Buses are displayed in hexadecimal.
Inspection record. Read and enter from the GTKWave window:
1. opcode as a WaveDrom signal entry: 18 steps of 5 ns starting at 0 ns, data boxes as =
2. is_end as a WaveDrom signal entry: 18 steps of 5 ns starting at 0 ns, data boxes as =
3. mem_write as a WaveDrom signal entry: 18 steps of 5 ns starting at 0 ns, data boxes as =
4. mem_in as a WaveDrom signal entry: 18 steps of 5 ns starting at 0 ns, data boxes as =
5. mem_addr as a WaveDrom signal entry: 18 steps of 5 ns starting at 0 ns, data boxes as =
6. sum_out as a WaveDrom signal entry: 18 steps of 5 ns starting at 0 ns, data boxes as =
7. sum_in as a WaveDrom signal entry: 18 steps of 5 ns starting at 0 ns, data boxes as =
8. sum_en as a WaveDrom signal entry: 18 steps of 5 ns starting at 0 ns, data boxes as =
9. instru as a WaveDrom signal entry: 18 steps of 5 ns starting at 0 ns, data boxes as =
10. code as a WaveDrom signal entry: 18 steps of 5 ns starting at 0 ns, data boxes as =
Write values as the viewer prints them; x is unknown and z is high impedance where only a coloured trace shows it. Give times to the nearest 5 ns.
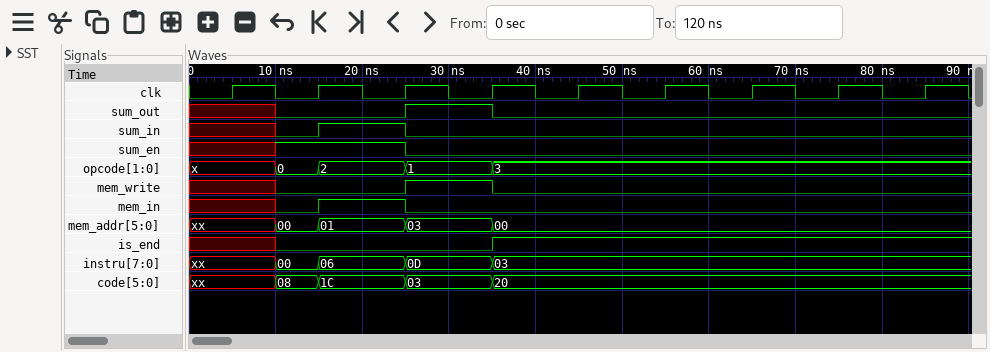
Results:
{name: 'opcode', wave: 'x.==.=.=..........', data: '0 2 1 3'}
{name: 'is_end', wave: 'x.0....1..........'}
{name: 'mem_write', wave: 'x.0..1.0..........'}
{name: 'mem_in', wave: 'x.01.0............'}
{name: 'mem_addr', wave: 'x.==.=.=..........', data: '00 01 03 00'}
{name: 'sum_out', wave: 'x.0..1.0..........'}
{name: 'sum_in', wave: 'x.01.0............'}
{name: 'sum_en', wave: 'x.1..0............'}
{name: 'instru', wave: 'x.==.=.=..........', data: '00 06 0D 03'}
{name: 'code', wave: 'x.==.=.=..........', data: '08 1C 03 20'}
